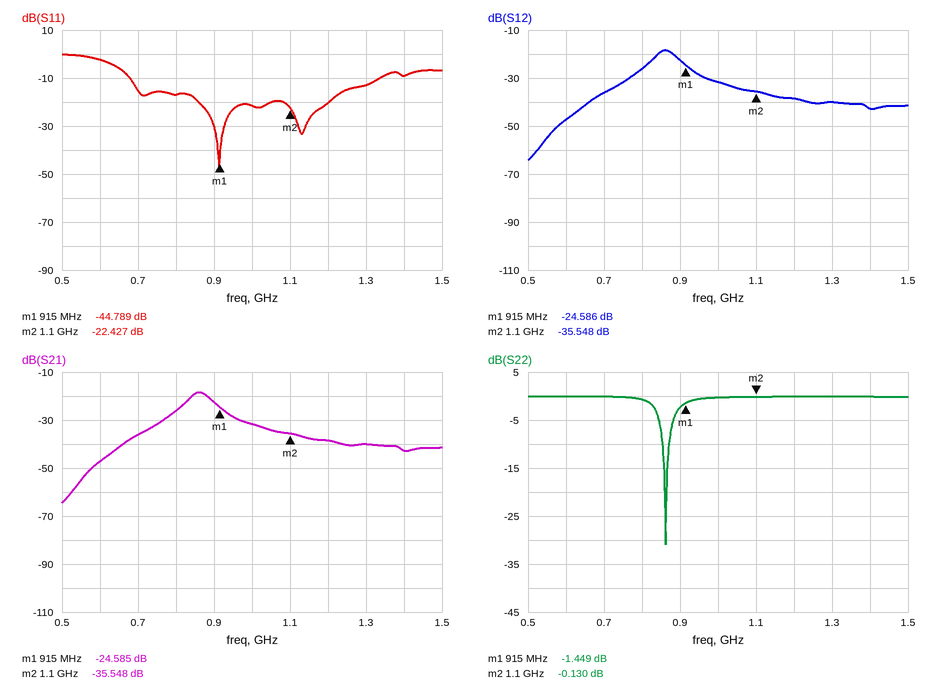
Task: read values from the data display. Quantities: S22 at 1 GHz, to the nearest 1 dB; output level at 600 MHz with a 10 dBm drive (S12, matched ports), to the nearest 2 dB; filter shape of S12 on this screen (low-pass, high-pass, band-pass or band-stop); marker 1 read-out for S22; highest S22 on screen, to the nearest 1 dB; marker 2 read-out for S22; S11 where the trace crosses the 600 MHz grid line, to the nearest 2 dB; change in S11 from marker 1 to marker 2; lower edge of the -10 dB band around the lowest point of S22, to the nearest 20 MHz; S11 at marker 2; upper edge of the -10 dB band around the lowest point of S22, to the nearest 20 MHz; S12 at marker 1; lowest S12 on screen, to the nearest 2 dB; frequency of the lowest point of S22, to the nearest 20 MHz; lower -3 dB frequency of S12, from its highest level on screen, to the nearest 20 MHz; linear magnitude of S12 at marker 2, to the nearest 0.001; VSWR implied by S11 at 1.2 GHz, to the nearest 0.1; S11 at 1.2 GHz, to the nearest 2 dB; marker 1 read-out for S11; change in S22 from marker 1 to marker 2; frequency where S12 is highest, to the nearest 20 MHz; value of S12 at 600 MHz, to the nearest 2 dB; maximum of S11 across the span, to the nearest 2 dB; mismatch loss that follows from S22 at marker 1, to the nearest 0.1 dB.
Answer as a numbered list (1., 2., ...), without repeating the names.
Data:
1. 0 dB
2. -38 dBm
3. band-pass
4. -1.449 dB
5. 0 dB
6. -0.130 dB
7. -2 dB
8. 22.362 dB
9. 860 MHz
10. -22.427 dB
11. 880 MHz
12. -24.586 dB
13. -64 dB
14. 860 MHz
15. 840 MHz
16. 0.017
17. 1.2
18. -20 dB
19. -44.789 dB
20. 1.319 dB
21. 860 MHz
22. -48 dB
23. 0 dB
24. 5.5 dB
